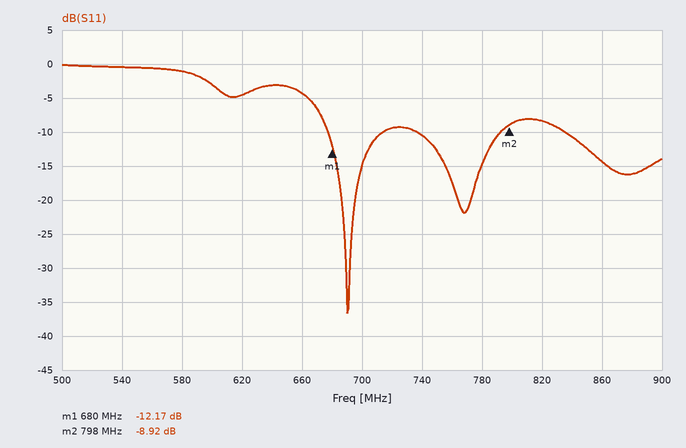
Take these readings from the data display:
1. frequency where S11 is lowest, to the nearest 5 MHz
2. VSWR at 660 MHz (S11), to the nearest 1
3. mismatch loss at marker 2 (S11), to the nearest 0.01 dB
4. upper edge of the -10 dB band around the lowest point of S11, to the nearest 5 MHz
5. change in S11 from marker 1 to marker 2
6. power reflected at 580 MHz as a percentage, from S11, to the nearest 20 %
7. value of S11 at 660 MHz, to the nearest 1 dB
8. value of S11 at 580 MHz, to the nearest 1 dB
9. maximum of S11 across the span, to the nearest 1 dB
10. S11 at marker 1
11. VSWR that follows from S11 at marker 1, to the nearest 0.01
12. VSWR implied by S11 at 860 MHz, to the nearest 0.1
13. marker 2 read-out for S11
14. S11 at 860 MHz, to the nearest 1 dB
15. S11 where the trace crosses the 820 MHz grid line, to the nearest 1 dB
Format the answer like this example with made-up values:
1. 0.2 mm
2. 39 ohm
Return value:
1. 690 MHz
2. 4
3. 0.60 dB
4. 715 MHz
5. 3.25 dB
6. 80 %
7. -4 dB
8. -1 dB
9. 0 dB
10. -12.17 dB
11. 1.65
12. 1.5
13. -8.92 dB
14. -14 dB
15. -8 dB
